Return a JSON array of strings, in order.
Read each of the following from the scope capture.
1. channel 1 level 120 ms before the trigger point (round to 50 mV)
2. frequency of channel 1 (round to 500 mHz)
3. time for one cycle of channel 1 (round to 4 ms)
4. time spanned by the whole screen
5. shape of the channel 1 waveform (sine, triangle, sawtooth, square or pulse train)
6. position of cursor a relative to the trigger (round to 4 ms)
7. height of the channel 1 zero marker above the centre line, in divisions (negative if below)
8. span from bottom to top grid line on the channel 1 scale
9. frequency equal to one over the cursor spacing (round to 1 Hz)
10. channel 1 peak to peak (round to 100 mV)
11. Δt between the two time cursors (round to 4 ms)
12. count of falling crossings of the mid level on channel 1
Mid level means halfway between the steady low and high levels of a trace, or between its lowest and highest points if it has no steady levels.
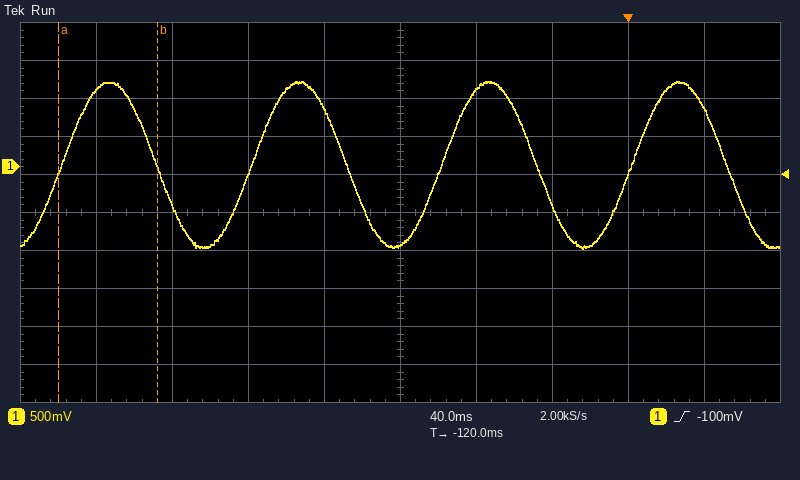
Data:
["-1.05 V", "10.0 Hz", "100 ms", "400 ms", "sine", "-300 ms", "+1.2 div", "5 V", "19 Hz", "2.20 V", "52 ms", "4"]
